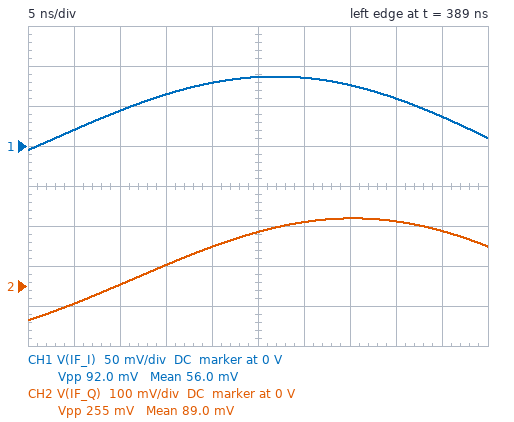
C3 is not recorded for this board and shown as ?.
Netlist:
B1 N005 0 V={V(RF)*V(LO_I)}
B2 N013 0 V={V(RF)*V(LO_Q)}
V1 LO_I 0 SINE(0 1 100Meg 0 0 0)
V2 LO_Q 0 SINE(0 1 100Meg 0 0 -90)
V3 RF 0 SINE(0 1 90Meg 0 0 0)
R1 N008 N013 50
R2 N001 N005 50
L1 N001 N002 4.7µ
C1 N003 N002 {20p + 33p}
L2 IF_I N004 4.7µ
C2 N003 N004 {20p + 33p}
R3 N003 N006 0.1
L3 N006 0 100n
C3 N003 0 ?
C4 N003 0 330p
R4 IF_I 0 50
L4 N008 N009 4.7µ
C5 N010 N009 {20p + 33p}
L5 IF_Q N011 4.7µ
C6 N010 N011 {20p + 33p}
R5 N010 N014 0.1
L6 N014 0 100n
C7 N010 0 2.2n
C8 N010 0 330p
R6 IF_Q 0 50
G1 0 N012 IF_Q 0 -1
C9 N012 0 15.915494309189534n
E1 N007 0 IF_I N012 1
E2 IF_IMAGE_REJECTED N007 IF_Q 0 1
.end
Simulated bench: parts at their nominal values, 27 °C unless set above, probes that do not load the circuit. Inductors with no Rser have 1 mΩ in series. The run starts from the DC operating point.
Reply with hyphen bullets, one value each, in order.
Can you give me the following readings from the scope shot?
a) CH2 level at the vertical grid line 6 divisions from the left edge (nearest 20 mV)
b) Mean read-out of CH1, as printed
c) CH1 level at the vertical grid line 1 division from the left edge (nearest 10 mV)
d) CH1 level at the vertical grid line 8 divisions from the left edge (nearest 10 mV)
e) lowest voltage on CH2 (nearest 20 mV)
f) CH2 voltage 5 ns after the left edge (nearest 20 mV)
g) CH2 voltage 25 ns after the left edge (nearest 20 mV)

- 160 mV
- 56.0 mV
- 20 mV
- 60 mV
- -80 mV
- -40 mV
- 140 mV
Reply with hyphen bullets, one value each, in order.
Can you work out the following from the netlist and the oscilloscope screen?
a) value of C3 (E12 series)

- 3.3 nF
